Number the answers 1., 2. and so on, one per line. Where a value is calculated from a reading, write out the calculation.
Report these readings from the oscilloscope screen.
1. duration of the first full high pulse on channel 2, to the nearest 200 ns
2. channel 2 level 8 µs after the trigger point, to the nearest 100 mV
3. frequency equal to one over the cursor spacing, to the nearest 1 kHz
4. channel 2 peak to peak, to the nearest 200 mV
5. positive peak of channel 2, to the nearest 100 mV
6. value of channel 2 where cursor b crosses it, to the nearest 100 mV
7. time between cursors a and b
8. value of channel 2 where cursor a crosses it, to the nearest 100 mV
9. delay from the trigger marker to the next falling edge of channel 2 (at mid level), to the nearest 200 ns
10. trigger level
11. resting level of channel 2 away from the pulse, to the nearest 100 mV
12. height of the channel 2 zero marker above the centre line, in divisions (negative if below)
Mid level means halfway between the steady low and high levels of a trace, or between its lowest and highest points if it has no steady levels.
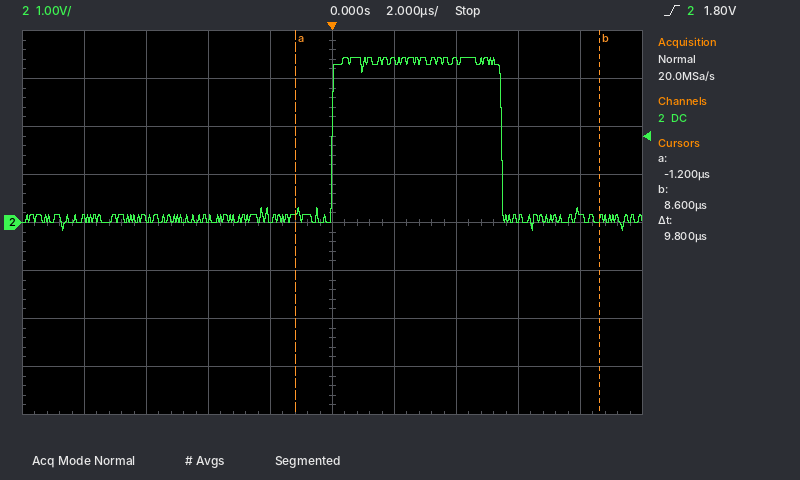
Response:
1. 5.4 µs
2. 200 mV
3. 1 / 9.8 µs ≈ 102 kHz
4. 3.6 V
5. 3.4 V
6. 100 mV
7. 9.8 µs
8. 200 mV
9. 5.4 µs
10. 1.80 V
11. 100 mV
12. 0.0 div
